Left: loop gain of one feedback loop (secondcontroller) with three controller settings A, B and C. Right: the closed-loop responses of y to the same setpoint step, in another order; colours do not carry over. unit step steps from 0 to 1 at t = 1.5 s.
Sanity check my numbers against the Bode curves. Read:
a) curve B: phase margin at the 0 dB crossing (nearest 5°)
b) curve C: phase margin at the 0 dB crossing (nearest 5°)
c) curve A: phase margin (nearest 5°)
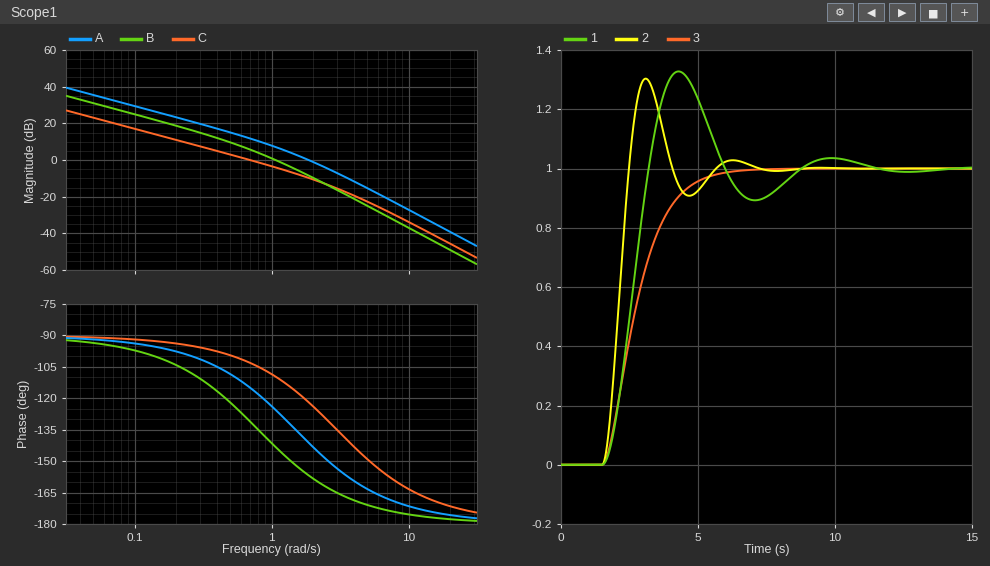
35°
75°
40°
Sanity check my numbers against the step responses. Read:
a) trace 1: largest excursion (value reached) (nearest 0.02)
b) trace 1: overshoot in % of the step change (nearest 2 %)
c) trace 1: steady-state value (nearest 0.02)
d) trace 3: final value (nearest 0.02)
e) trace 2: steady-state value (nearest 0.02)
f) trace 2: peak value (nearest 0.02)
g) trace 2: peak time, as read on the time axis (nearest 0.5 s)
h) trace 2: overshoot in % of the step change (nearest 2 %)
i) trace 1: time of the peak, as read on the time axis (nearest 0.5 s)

1.32
32 %
1.00
1.00
1.00
1.30
3.0 s
30 %
4.5 s
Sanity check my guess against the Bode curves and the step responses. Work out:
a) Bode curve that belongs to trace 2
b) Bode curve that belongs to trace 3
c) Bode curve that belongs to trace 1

A
C
B
